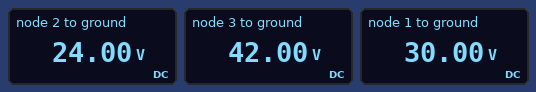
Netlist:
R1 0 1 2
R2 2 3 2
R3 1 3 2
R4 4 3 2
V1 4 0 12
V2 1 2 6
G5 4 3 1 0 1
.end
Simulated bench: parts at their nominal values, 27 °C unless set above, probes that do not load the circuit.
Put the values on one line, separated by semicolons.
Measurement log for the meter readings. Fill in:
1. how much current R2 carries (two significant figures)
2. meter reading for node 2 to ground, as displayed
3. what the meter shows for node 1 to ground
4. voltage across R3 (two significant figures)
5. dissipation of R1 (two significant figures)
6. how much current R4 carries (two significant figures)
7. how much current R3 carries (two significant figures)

9.0 A; 24.00 V; 30.00 V; 12 V; 450 W; 15 A; 6.0 A
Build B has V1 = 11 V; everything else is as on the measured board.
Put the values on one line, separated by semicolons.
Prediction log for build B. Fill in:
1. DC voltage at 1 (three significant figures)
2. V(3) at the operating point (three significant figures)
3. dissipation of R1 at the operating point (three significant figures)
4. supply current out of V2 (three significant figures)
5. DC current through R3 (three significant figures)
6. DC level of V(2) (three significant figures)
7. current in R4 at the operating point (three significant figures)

28.0 V; 39.0 V; 392 W; 8.50 A; 5.50 A; 22.0 V; 14.0 A
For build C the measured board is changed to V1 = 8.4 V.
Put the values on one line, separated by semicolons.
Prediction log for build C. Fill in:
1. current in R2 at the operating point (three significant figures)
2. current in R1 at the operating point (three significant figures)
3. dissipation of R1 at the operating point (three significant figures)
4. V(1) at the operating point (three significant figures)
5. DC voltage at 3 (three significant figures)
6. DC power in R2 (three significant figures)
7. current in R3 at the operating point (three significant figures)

7.20 A; 11.4 A; 260 W; 22.8 V; 31.2 V; 104 W; 4.20 A
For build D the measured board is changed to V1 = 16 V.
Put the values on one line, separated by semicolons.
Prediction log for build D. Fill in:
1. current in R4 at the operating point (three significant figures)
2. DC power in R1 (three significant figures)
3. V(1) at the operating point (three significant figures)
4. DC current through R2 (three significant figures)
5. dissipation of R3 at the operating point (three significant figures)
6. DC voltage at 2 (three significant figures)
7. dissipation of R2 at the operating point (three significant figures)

19.0 A; 722 W; 38.0 V; 11.0 A; 128 W; 32.0 V; 242 W
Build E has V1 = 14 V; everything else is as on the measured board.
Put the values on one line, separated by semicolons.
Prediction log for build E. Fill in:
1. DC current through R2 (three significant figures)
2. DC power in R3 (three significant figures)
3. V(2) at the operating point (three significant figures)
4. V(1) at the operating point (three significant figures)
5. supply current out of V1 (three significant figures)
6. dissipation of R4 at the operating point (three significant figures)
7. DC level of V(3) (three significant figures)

10.0 A; 98.0 W; 28.0 V; 34.0 V; 17.0 A; 578 W; 48.0 V
